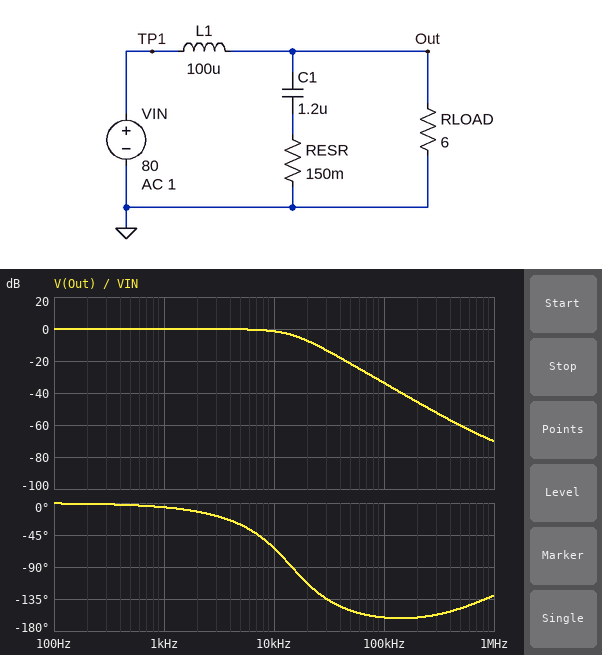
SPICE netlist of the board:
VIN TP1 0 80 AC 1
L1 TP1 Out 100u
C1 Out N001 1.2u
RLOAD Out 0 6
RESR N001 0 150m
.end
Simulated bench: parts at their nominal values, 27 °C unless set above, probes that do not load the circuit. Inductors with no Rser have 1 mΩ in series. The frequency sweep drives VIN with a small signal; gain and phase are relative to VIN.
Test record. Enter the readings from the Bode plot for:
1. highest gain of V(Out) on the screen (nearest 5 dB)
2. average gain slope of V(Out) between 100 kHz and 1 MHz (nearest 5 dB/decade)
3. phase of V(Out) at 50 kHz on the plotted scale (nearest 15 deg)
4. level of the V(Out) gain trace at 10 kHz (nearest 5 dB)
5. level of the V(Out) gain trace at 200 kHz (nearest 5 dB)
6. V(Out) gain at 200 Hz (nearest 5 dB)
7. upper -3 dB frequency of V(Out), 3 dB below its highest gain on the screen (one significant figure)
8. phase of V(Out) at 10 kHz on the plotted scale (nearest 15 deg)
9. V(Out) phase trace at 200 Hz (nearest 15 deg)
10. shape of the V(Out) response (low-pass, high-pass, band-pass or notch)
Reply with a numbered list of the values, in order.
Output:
1. 0 dB
2. -35 dB/decade
3. -150 deg
4. 0 dB
5. -45 dB
6. 0 dB
7. 10 kHz
8. -60 deg
9. 0 deg
10. low-pass
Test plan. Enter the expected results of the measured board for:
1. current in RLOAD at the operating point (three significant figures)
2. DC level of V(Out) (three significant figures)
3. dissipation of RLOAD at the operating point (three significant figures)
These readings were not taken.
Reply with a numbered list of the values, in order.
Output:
1. 13.3 A
2. 80.0 V
3. 1.07 kW
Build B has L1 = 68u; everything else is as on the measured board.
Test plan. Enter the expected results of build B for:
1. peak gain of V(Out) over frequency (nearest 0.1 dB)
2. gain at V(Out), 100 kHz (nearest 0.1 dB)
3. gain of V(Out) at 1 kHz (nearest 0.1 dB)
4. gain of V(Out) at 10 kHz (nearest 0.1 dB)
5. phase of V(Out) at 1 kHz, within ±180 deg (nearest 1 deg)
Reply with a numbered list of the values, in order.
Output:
1. 0.2 dB
2. -30.3 dB
3. 0 dB
4. 0.1 dB
5. -4 deg
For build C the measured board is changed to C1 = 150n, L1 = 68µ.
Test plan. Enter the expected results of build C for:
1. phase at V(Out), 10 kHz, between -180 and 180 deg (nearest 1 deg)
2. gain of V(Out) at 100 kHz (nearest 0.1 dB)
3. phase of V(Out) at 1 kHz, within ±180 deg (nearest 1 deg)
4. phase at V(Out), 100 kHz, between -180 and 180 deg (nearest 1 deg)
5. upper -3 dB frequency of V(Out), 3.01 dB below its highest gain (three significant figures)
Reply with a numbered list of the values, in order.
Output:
1. -37 deg
2. -17.8 dB
3. -4 deg
4. -113 deg
5. 15.2 kHz
